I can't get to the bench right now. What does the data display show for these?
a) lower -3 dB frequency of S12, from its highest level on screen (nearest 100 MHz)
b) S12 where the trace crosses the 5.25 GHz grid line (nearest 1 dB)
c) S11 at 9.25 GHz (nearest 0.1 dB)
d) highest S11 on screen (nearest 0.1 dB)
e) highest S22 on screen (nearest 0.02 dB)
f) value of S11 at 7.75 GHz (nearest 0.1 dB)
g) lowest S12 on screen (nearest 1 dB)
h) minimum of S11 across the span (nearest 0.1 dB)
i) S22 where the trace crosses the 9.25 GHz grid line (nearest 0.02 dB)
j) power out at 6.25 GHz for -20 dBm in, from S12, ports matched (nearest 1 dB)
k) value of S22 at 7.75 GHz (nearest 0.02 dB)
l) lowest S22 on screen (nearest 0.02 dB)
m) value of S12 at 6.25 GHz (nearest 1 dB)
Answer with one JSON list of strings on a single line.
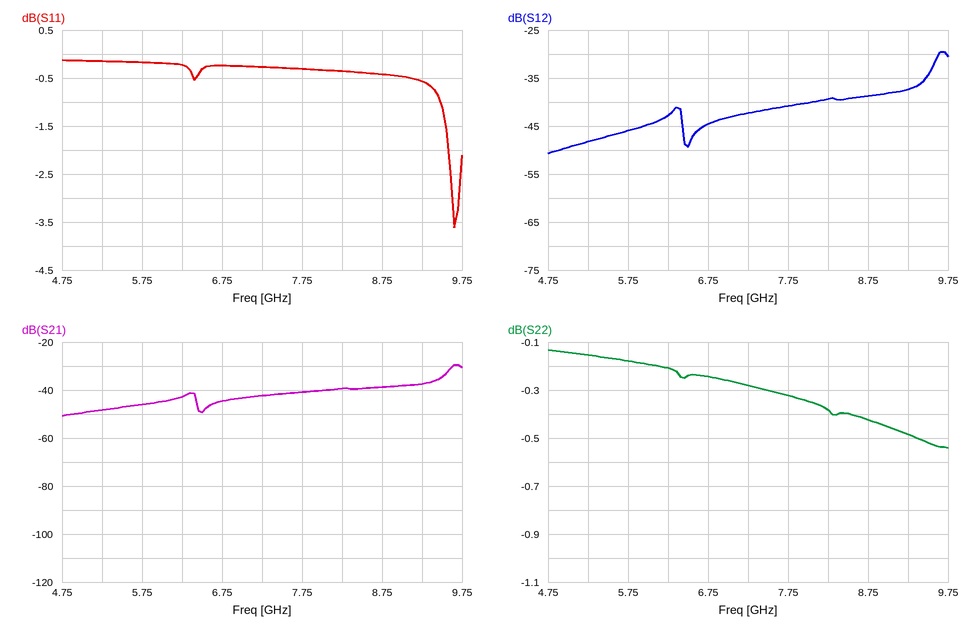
["9.6 GHz", "-48 dB", "-0.6 dB", "-0.1 dB", "-0.14 dB", "-0.3 dB", "-51 dB", "-3.6 dB", "-0.48 dB", "-63 dBm", "-0.32 dB", "-0.54 dB", "-43 dB"]
